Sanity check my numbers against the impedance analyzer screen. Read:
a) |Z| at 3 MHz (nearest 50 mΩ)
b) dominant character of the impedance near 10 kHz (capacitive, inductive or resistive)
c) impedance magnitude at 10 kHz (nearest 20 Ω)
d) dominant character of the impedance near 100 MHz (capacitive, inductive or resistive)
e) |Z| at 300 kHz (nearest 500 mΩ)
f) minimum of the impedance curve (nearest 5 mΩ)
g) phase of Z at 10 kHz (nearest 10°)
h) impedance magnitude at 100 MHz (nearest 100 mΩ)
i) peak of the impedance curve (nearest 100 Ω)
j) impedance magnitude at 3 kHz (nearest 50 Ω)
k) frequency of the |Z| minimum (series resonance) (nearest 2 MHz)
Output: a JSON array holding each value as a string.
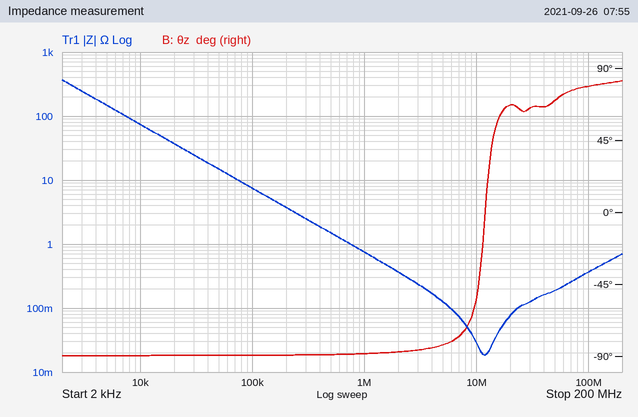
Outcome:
["250 mΩ", "capacitive", "80 Ω", "inductive", "2.5 Ω", "20 mΩ", "-90°", "400 mΩ", "400 Ω", "250 Ω", "12 MHz"]
